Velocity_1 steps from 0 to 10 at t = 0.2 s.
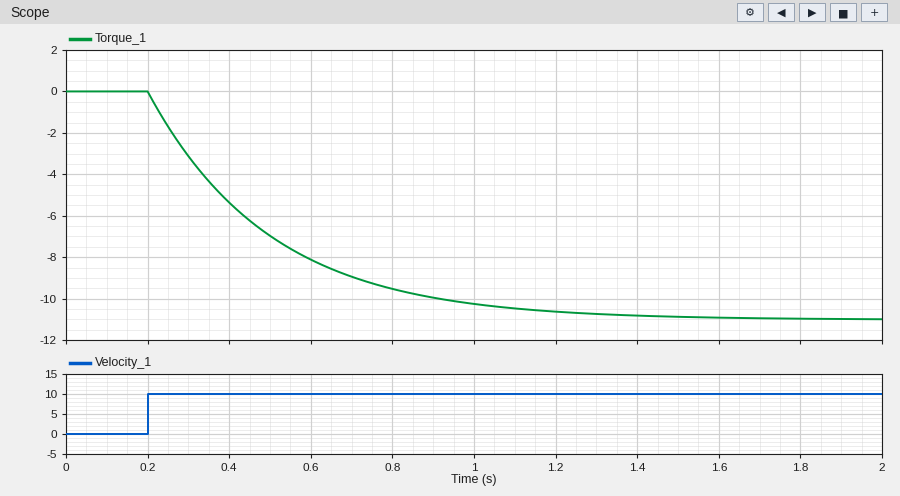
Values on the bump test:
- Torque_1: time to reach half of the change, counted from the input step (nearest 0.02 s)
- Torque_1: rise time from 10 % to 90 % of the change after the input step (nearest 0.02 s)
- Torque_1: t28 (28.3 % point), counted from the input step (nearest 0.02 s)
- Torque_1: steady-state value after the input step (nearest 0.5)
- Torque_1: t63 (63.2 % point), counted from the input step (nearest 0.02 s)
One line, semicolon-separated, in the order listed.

0.20 s; 0.66 s; 0.10 s; -11.0; 0.30 s
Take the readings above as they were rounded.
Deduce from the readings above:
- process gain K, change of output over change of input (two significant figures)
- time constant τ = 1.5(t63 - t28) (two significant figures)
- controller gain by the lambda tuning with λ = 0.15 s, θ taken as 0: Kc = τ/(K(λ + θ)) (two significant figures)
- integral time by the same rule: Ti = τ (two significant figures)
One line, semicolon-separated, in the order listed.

-1.1; 0.30 s; -1.8; 0.30 s
